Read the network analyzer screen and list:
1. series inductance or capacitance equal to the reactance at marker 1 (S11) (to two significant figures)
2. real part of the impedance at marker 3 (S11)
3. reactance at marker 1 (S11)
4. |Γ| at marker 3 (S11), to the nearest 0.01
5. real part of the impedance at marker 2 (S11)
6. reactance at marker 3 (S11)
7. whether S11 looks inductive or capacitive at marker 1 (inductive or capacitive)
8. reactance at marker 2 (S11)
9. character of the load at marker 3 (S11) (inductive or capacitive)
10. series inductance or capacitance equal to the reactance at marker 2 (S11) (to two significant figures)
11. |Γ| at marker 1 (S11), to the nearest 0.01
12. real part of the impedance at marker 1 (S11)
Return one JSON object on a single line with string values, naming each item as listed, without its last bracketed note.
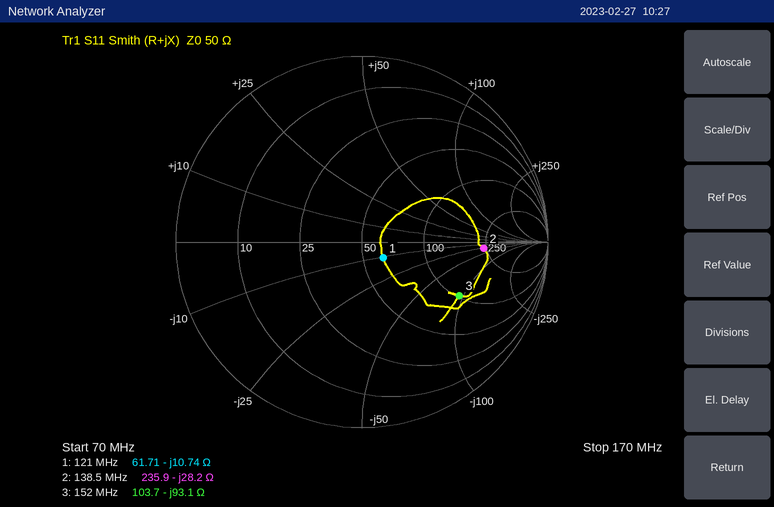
{"series inductance or capacitance equal to the reactance at marker 1 (S11)": "120 pF", "real part of the impedance at marker 3": "103.7 Ω", "reactance at marker 1": "-10.74 Ω", "|Γ| at marker 3 (S11), to the nearest 0.01": "0.60", "real part of the impedance at marker 2": "235.9 Ω", "reactance at marker 3": "-93.1 Ω", "whether S11 looks inductive or capacitive at marker 1": "capacitive", "reactance at marker 2": "-28.2 Ω", "character of the load at marker 3 (S11)": "capacitive", "series inductance or capacitance equal to the reactance at marker 2 (S11)": "41 pF", "|Γ| at marker 1 (S11), to the nearest 0.01": "0.14", "real part of the impedance at marker 1": "61.71 Ω"}
